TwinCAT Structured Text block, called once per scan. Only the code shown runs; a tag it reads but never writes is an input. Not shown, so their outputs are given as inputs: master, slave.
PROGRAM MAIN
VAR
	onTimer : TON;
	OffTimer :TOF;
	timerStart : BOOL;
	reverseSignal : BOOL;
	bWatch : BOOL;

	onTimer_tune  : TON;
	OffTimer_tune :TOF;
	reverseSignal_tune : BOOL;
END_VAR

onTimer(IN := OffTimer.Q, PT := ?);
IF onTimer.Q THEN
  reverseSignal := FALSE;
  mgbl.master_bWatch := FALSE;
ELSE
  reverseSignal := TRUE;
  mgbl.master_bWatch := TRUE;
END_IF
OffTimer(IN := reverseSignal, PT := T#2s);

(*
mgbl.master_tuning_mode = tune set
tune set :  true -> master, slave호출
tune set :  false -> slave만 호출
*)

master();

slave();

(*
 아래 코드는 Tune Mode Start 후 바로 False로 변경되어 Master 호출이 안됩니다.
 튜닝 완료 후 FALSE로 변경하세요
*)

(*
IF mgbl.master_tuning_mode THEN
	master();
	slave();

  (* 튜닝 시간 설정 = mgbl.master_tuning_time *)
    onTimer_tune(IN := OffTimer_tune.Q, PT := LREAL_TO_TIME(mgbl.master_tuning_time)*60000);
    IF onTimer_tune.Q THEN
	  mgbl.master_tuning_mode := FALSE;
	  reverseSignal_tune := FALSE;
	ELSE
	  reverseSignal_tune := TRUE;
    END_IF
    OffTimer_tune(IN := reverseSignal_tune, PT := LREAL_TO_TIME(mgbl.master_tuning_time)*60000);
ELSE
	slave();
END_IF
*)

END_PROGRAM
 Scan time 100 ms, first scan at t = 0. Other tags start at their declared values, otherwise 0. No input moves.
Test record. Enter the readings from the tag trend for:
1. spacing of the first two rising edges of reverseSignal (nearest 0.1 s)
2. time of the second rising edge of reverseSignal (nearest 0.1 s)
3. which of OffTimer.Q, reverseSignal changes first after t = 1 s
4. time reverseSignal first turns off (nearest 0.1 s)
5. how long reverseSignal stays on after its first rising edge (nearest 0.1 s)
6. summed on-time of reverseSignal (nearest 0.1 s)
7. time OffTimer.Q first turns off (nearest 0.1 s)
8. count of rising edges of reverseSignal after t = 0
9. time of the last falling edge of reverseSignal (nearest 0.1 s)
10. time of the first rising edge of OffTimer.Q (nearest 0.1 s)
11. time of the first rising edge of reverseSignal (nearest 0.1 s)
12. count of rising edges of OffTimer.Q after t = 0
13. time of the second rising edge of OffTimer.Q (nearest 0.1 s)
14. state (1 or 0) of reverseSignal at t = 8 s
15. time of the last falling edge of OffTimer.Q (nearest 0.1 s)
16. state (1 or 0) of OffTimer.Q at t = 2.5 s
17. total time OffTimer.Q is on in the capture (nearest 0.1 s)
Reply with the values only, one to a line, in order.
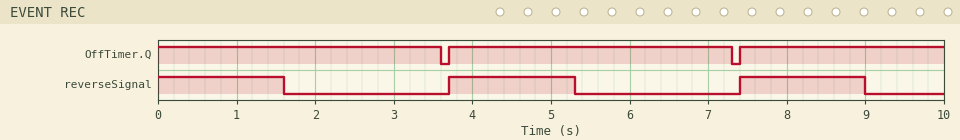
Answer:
3.7 s
7.4 s
reverseSignal
1.6 s
1.6 s
4.8 s
3.6 s
2
9.0 s
3.7 s
3.7 s
2
7.4 s
1
7.3 s
1
9.8 s
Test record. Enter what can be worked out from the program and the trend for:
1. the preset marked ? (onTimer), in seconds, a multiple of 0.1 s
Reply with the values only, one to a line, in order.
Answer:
1.5 s
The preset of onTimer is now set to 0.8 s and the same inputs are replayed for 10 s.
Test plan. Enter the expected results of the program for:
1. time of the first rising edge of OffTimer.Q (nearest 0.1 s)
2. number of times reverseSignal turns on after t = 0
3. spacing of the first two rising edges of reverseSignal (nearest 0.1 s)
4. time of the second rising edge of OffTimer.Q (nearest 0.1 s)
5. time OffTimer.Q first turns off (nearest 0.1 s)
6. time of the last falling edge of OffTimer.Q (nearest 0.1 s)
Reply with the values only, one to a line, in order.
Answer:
3.0 s
3
3.0 s
6.0 s
2.9 s
8.9 s
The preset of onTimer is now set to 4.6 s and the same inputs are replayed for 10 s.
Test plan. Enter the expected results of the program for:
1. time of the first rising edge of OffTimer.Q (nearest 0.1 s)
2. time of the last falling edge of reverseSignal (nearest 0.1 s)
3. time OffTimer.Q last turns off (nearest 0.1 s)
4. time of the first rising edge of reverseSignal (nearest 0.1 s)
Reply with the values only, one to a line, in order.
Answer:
6.8 s
4.7 s
6.7 s
6.8 s
